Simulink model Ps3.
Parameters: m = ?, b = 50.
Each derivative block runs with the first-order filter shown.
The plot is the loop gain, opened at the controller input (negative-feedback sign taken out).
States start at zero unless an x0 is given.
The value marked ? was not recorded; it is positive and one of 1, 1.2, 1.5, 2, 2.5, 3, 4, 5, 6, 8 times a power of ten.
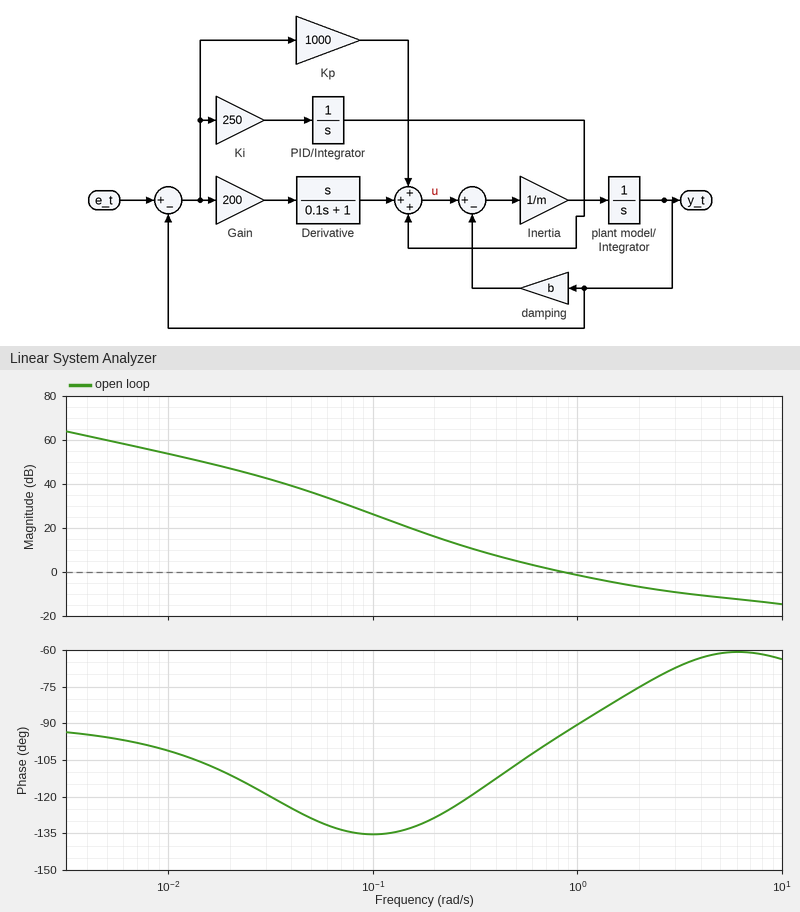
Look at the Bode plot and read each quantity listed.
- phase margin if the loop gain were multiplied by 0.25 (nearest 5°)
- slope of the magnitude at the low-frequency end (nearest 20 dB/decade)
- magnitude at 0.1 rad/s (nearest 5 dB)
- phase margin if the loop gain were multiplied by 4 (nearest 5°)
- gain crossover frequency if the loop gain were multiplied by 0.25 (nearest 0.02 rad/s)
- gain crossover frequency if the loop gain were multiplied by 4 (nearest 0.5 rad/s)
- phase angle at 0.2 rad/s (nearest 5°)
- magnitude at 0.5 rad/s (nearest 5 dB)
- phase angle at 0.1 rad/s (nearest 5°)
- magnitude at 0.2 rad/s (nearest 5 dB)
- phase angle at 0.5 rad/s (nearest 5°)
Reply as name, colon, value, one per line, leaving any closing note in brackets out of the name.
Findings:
phase margin if the loop gain were multiplied by 0.25: 60°
slope of the magnitude at the low-frequency end: -20 dB/decade
magnitude at 0.1 rad/s: 25 dB
phase margin if the loop gain were multiplied by 4: 120°
gain crossover frequency if the loop gain were multiplied by 0.25: 0.28 rad/s
gain crossover frequency if the loop gain were multiplied by 4: 5.5 rad/s
phase angle at 0.2 rad/s: -130°
magnitude at 0.5 rad/s: 5 dB
phase angle at 0.1 rad/s: -135°
magnitude at 0.2 rad/s: 15 dB
phase angle at 0.5 rad/s: -105°
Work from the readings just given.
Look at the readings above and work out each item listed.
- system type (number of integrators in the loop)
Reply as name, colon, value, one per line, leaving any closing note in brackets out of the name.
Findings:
system type: 1
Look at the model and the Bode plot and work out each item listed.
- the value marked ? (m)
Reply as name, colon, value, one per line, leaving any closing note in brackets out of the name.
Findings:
the value marked ?: 1200
